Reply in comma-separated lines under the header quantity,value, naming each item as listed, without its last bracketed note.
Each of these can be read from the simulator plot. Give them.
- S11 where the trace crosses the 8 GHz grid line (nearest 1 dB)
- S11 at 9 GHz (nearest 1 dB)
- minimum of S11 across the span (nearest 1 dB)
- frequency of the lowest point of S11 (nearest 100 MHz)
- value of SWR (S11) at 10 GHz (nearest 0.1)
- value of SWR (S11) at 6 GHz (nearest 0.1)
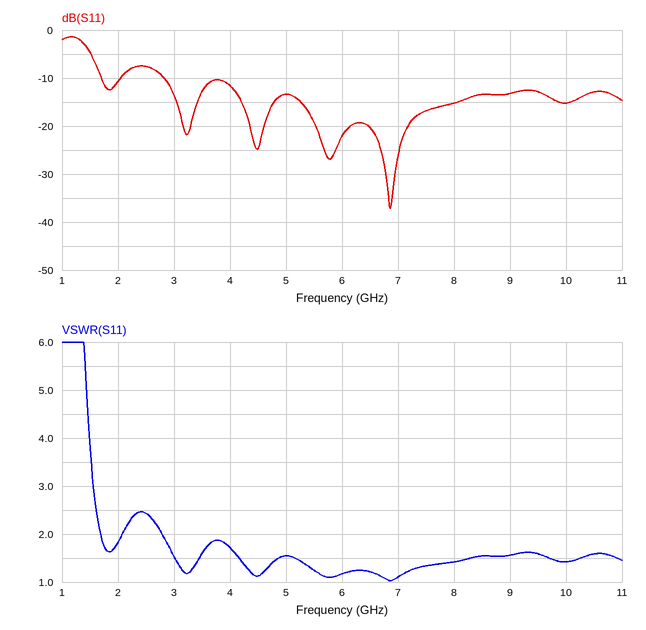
quantity,value
S11 where the trace crosses the 8 GHz grid line,-15 dB
S11 at 9 GHz,-13 dB
minimum of S11 across the span,-37 dB
frequency of the lowest point of S11,6.9 GHz
value of SWR (S11) at 10 GHz,1.4
value of SWR (S11) at 6 GHz,1.2
